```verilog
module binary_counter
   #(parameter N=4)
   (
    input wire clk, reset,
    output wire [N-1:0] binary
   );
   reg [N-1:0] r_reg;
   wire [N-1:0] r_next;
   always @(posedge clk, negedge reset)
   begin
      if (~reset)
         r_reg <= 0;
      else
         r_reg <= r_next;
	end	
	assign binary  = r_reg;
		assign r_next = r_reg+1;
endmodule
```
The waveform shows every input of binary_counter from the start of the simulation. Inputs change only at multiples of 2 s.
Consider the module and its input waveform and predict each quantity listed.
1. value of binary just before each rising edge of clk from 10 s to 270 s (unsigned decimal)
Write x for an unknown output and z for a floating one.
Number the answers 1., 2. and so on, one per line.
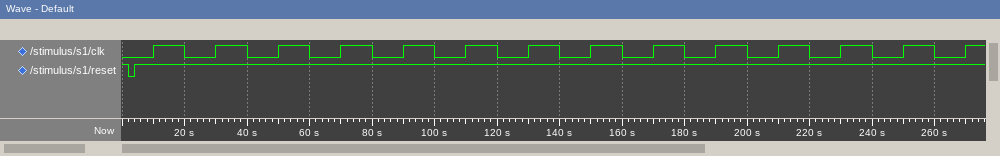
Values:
1. 0, 1, 2, 3, 4, 5, 6, 7, 8, 9, 10, 11, 12, 13
